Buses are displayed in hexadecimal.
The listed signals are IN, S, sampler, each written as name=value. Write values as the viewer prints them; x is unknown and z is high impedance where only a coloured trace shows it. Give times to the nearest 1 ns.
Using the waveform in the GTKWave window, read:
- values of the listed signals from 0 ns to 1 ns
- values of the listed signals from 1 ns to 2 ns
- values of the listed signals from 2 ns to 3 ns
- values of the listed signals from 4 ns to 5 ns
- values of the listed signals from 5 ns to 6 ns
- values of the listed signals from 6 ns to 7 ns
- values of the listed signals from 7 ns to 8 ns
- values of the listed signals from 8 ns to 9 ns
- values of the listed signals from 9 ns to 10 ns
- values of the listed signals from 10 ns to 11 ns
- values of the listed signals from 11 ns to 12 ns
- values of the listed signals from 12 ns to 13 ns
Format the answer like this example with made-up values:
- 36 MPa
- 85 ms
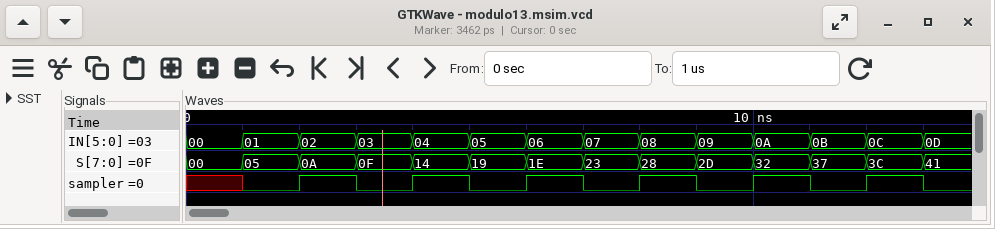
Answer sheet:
- IN=00, S=00, sampler=x
- IN=01, S=05, sampler=0
- IN=02, S=0A, sampler=1
- IN=04, S=14, sampler=1
- IN=05, S=19, sampler=0
- IN=06, S=1E, sampler=1
- IN=07, S=23, sampler=0
- IN=08, S=28, sampler=1
- IN=09, S=2D, sampler=0
- IN=0A, S=32, sampler=1
- IN=0B, S=37, sampler=0
- IN=0C, S=3C, sampler=1
